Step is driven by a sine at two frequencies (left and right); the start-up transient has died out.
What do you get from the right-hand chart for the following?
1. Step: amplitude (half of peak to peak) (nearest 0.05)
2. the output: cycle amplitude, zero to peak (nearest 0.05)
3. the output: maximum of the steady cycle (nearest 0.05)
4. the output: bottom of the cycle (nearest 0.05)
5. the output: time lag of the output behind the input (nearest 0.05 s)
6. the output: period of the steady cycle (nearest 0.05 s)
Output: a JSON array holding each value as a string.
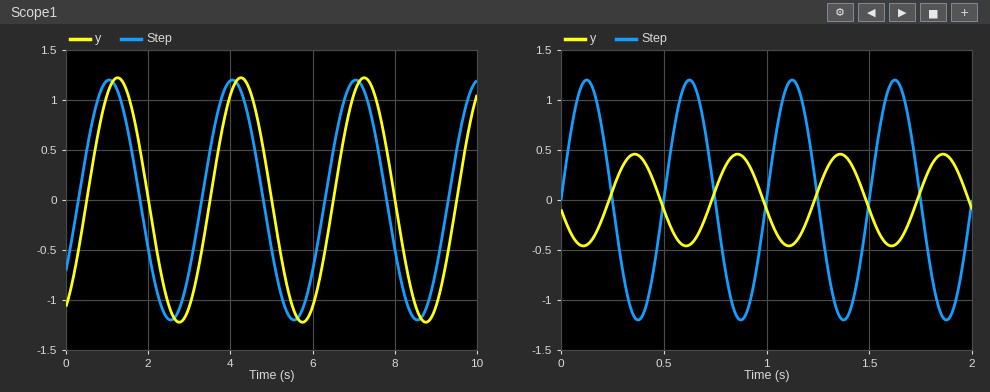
["1.20", "0.45", "0.45", "-0.45", "0.25 s", "0.50 s"]
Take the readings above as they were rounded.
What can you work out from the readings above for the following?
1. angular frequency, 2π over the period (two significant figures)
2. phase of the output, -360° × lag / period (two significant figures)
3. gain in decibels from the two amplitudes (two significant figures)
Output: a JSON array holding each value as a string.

["13 rad/s", "-180°", "-8.5 dB"]
